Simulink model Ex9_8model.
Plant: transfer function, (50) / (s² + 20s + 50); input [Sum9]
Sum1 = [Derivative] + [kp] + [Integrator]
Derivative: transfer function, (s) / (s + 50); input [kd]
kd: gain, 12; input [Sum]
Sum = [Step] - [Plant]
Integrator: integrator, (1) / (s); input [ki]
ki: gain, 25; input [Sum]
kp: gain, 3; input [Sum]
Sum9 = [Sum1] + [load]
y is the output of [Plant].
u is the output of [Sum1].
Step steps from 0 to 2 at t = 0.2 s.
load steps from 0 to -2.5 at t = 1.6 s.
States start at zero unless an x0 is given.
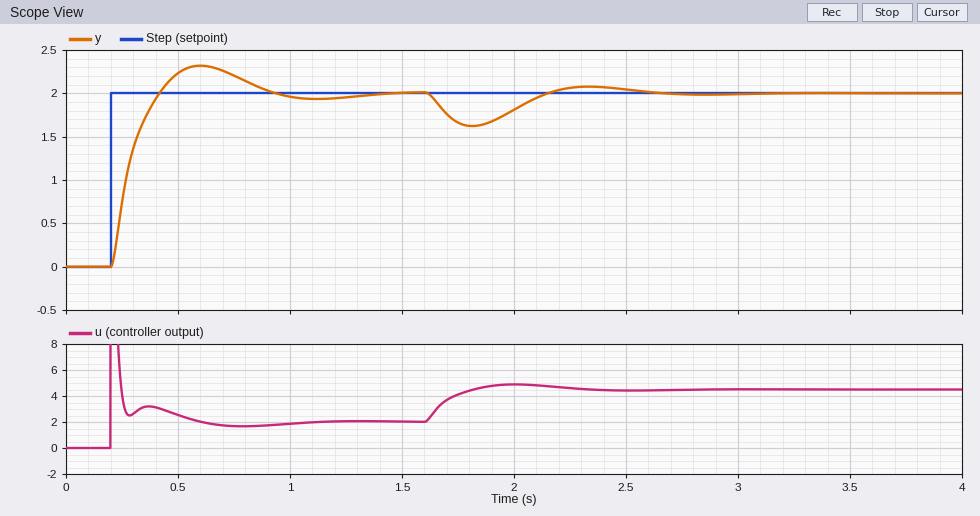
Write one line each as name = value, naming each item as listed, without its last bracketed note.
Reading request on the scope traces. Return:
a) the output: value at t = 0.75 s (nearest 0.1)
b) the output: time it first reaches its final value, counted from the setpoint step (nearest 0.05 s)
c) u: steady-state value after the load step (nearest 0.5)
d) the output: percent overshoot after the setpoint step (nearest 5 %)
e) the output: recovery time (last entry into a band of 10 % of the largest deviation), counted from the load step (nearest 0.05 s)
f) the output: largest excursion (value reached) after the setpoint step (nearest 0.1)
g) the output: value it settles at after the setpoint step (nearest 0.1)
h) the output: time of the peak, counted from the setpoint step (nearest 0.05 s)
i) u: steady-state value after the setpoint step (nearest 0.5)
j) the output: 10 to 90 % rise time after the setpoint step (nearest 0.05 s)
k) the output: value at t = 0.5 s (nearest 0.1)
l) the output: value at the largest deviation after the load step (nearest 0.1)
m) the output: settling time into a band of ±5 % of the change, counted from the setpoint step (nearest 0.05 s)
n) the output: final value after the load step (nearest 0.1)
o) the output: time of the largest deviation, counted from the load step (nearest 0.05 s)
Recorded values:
the output: value at t = 0.75 s = 2.2
the output: time it first reaches its final value, counted from the setpoint step = 0.20 s
u: steady-state value after the load step = 4.5
the output: percent overshoot after the setpoint step = 15 %
the output: recovery time (last entry into a band of 10 % of the largest deviation), counted from the load step = 0.90 s
the output: largest excursion (value reached) after the setpoint step = 2.3
the output: value it settles at after the setpoint step = 2.0
the output: time of the peak, counted from the setpoint step = 0.40 s
u: steady-state value after the setpoint step = 2.0
the output: 10 to 90 % rise time after the setpoint step = 0.15 s
the output: value at t = 0.5 s = 2.2
the output: value at the largest deviation after the load step = 1.6
the output: settling time into a band of ±5 % of the change, counted from the setpoint step = 0.65 s
the output: final value after the load step = 2.0
the output: time of the largest deviation, counted from the load step = 0.20 s
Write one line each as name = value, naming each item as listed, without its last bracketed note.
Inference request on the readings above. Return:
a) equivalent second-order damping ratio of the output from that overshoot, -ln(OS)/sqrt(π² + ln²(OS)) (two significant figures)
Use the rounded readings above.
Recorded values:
equivalent second-order damping ratio of the output from that overshoot, -ln(OS)/sqrt(π² + ln²(OS)) = 0.52
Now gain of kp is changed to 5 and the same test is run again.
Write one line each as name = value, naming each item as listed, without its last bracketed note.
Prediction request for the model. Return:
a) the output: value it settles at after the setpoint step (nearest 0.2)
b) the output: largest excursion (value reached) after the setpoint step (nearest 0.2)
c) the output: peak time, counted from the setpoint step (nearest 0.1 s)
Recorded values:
the output: value it settles at after the setpoint step = 2.0
the output: largest excursion (value reached) after the setpoint step = 2.2
the output: peak time, counted from the setpoint step = 0.3 s
